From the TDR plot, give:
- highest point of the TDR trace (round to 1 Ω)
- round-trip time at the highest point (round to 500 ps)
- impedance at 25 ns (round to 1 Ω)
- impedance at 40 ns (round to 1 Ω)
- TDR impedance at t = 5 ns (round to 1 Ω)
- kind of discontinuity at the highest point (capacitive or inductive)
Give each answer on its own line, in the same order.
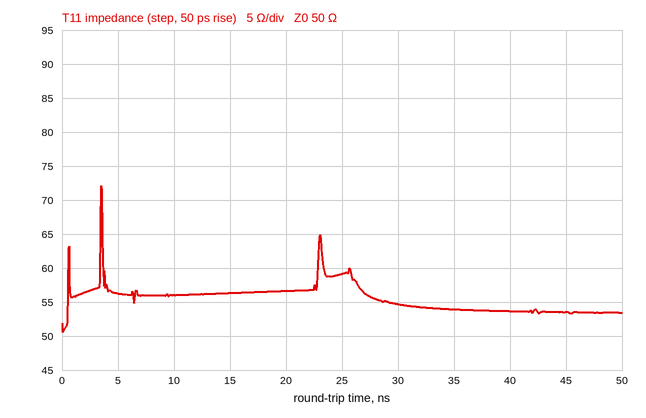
72 Ω
3.5 ns
59 Ω
54 Ω
56 Ω
inductive
